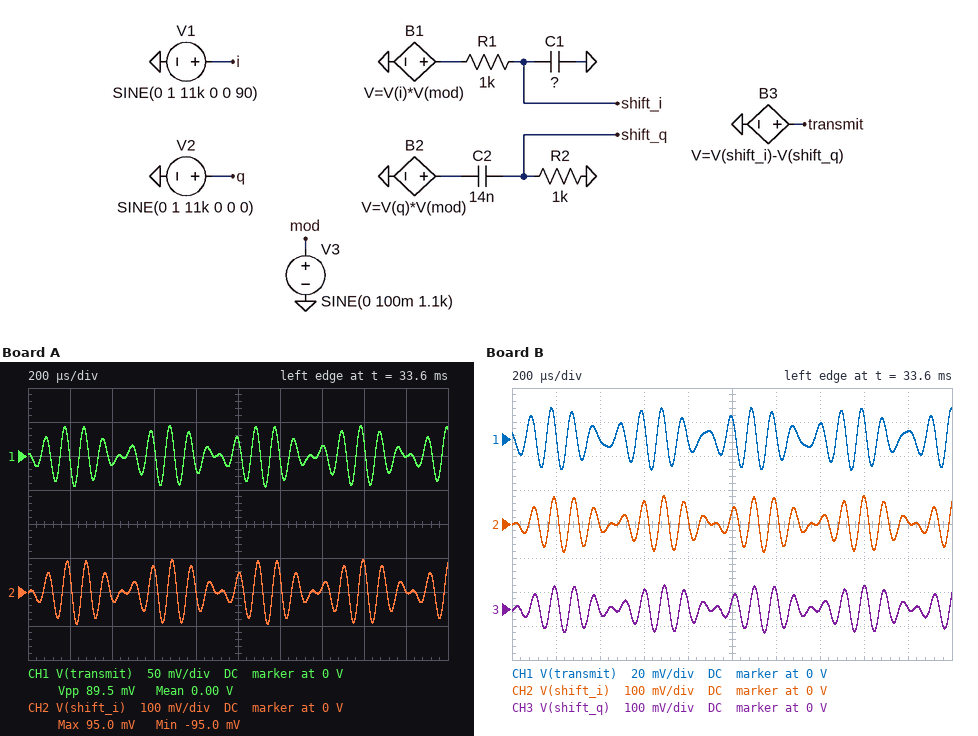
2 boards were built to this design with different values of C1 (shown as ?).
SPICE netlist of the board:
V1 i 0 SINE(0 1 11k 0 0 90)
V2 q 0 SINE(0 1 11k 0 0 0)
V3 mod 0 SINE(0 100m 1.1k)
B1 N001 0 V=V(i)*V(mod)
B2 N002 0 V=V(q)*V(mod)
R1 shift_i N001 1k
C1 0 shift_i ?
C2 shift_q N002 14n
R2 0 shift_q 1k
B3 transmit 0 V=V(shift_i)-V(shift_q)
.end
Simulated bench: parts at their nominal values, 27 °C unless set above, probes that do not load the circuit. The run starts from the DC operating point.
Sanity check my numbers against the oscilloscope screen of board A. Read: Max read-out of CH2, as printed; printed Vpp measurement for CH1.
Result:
95.0 mV
89.5 mV
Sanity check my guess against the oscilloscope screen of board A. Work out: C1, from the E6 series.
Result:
4.7 nF
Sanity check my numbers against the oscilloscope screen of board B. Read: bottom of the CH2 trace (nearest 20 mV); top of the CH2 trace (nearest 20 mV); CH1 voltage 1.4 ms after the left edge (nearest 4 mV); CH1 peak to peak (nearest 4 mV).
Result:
-80 mV
80 mV
8 mV
36 mV
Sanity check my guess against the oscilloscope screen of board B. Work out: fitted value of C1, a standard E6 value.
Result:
10 nF
